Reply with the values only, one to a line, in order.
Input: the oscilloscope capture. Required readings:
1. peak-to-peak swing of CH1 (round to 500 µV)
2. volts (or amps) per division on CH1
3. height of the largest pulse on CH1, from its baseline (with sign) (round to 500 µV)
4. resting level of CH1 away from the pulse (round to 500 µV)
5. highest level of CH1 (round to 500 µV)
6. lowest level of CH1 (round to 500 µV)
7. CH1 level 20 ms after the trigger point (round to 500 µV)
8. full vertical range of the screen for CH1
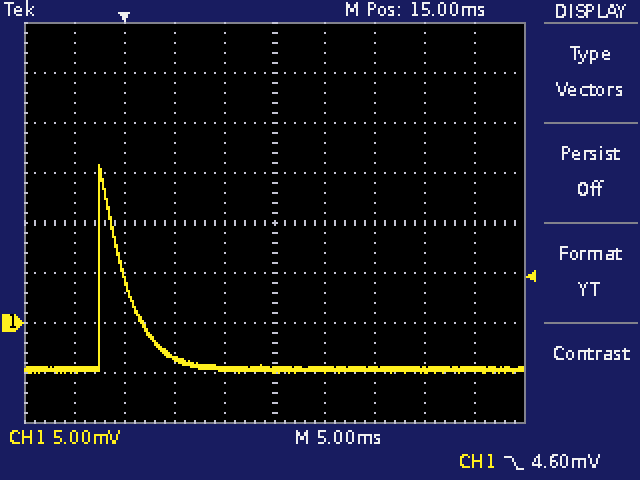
21.0 mV
5 mV
+20.5 mV
-4.5 mV
16.0 mV
-5.0 mV
-4.5 mV
40 mV
